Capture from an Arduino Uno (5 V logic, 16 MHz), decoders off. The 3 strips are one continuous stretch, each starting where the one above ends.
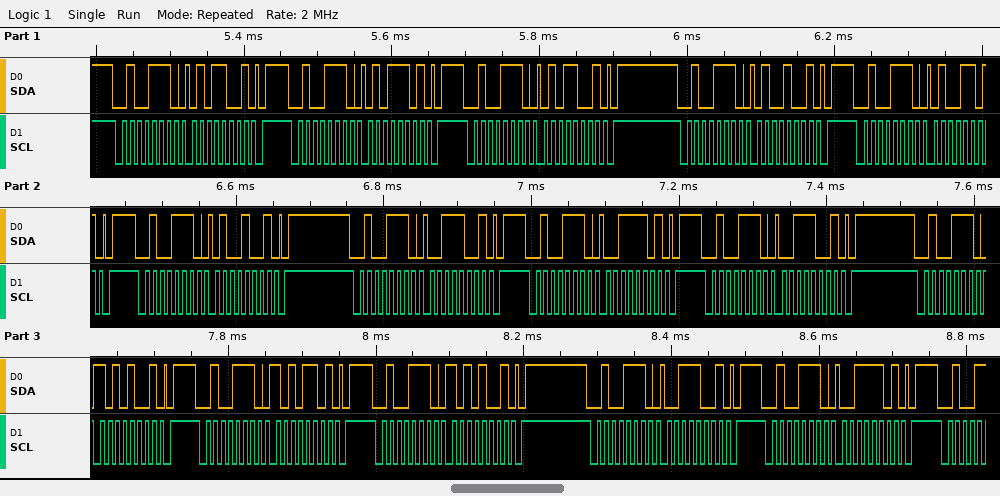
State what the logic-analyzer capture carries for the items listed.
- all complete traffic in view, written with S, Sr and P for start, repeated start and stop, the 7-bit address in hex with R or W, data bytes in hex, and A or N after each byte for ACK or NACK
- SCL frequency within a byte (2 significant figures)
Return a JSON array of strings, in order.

["S 27W A 59 A P S 27W A 5D A P S 27W A 59 A P S 27W A 49 A P S 27W A 4D A P S 27W A 49 A P S 27W A 39 A P S 27W A 3D A P S 27W A 39 A P S 27W A A9 A P S 27W A AD A P S 27W A A9 A P S 27W A 39 A P S 27W A 3D A P", "100 kHz"]
